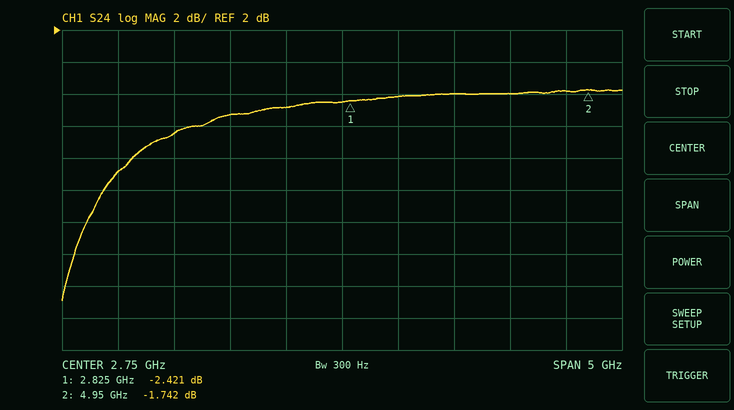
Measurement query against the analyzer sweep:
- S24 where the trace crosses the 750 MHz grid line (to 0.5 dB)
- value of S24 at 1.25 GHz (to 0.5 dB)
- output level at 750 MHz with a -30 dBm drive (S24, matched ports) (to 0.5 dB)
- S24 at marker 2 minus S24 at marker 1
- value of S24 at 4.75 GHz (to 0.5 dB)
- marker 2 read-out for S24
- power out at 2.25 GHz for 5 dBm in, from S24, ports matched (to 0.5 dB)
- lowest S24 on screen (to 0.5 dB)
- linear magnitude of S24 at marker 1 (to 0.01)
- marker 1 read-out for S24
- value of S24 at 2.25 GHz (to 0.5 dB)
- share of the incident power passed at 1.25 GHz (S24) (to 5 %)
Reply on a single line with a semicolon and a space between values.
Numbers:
-7.0 dB; -4.5 dB; -37.0 dBm; 0.679 dB; -2.0 dB; -1.742 dB; 2.0 dBm; -15.0 dB; 0.76; -2.421 dB; -3.0 dB; 35 %
